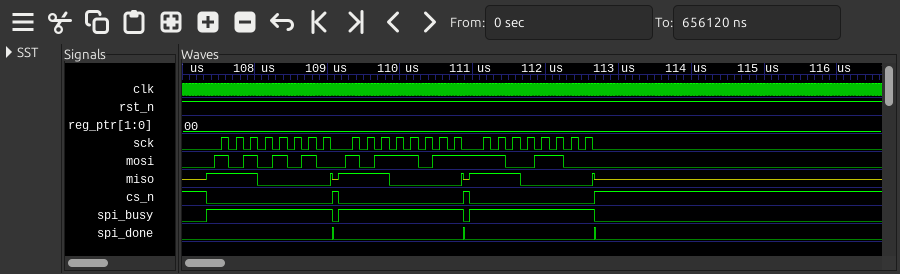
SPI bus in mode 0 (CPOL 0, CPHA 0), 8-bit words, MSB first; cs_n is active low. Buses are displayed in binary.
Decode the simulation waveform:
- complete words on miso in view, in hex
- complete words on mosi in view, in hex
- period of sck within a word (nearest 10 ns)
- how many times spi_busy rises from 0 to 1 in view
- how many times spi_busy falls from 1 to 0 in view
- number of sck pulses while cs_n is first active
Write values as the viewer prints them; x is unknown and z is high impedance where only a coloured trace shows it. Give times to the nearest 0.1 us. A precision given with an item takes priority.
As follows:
E0, E0, E0
AA, BB, CC
200 ns
3
3
8
